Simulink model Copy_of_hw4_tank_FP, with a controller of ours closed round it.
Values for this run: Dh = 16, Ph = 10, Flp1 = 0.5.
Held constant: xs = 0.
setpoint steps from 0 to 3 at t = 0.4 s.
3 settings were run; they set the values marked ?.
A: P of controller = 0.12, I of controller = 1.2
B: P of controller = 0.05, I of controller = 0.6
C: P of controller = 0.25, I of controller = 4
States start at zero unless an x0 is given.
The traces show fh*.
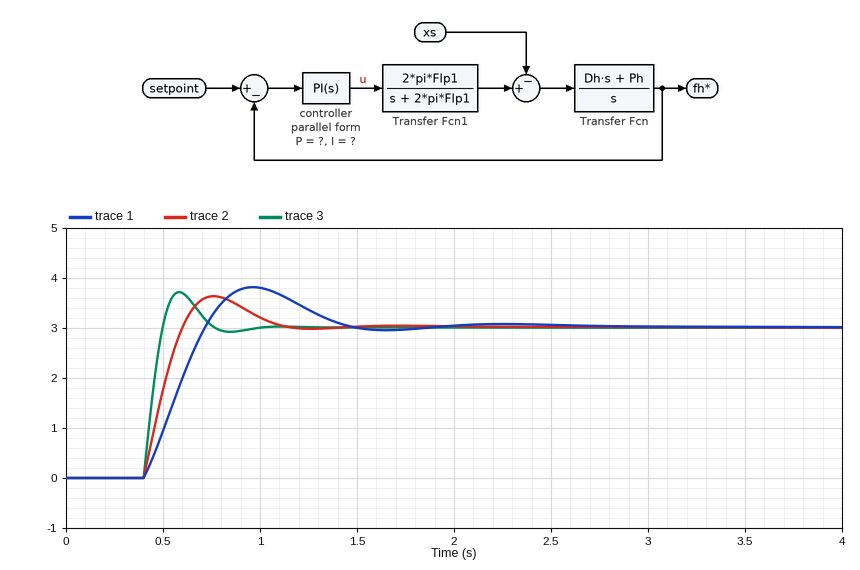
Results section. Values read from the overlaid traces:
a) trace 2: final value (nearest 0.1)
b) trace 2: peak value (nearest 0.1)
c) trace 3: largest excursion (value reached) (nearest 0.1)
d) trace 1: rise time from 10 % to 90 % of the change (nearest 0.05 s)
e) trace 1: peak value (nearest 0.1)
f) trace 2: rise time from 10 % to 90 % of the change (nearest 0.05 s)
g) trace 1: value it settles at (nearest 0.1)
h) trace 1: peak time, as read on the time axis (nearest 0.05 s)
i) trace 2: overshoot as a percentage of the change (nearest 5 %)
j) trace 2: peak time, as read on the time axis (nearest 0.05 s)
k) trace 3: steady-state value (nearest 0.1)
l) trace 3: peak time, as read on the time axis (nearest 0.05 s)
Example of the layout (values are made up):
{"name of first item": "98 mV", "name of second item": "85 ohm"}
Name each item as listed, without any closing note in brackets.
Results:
{"trace 2: final value": "3.0", "trace 2: peak value": "3.6", "trace 3: largest excursion (value reached)": "3.7", "trace 1: rise time from 10 % to 90 % of the change": "0.25 s", "trace 1: peak value": "3.8", "trace 2: rise time from 10 % to 90 % of the change": "0.15 s", "trace 1: value it settles at": "3.0", "trace 1: peak time, as read on the time axis": "0.95 s", "trace 2: overshoot as a percentage of the change": "20 %", "trace 2: peak time, as read on the time axis": "0.75 s", "trace 3: steady-state value": "3.0", "trace 3: peak time, as read on the time axis": "0.60 s"}
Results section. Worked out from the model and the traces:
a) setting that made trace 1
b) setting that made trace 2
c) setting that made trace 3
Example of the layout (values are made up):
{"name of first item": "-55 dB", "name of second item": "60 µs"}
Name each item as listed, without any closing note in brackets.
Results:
{"setting that made trace 1": "B", "setting that made trace 2": "A", "setting that made trace 3": "C"}
